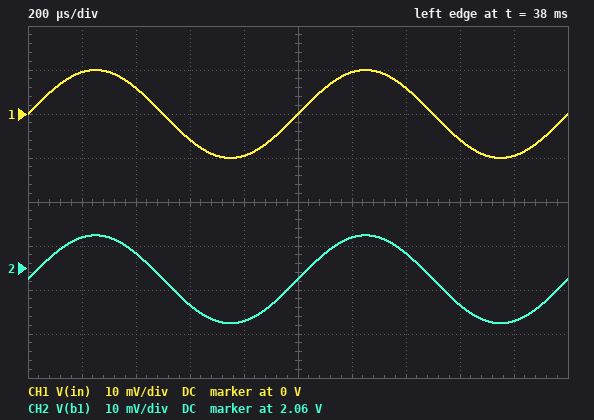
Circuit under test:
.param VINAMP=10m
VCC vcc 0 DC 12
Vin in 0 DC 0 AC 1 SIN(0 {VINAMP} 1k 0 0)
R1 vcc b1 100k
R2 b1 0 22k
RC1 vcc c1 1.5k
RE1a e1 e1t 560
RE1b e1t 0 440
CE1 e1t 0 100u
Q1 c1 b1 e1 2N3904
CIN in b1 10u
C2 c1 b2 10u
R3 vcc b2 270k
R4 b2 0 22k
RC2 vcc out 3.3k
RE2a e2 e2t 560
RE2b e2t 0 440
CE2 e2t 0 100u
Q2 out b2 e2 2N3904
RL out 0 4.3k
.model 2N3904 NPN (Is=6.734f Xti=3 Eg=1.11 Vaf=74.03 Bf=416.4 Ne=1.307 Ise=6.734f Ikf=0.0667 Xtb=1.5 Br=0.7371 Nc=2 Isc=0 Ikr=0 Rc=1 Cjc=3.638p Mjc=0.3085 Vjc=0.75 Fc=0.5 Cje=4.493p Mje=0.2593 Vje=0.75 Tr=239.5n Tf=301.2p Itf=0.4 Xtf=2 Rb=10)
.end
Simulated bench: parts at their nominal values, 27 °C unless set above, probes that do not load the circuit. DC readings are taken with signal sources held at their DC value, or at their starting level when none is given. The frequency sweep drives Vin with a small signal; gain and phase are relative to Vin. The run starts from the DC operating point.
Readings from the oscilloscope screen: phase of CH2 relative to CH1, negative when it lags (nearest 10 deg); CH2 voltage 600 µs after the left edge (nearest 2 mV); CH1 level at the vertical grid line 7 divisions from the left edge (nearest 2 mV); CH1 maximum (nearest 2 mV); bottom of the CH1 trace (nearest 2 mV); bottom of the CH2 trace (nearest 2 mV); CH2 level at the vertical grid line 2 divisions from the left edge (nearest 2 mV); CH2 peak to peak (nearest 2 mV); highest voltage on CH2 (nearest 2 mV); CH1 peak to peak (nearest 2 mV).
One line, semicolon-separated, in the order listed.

0 deg; 2.052 V; 6 mV; 10 mV; -10 mV; 2.048 V; 2.064 V; 20 mV; 2.068 V; 20 mV
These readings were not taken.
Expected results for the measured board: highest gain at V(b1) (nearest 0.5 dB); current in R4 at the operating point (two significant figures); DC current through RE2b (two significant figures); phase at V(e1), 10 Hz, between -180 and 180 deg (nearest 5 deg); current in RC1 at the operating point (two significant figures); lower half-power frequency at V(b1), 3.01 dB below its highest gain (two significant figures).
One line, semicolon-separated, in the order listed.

0 dB; 40 µA; 250 µA; 5 deg; 1.4 mA; 950 mHz
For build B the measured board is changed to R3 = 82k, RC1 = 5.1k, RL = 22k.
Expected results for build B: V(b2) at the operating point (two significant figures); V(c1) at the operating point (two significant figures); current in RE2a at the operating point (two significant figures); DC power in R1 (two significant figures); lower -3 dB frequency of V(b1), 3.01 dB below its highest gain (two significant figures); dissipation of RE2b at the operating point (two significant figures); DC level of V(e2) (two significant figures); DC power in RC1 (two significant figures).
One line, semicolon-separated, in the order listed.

2.4 V; 5.0 V; 1.7 mA; 990 µW; 960 mHz; 1.3 mW; 1.7 V; 9.6 mW
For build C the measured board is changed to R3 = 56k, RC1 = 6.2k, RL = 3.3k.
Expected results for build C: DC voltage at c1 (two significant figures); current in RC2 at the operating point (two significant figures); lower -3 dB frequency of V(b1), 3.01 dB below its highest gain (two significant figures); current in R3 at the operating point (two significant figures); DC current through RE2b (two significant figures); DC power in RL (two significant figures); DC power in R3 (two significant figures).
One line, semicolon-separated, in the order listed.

3.5 V; 2.9 mA; 960 mHz; 160 µA; 2.2 mA; 1.7 mW; 1.5 mW
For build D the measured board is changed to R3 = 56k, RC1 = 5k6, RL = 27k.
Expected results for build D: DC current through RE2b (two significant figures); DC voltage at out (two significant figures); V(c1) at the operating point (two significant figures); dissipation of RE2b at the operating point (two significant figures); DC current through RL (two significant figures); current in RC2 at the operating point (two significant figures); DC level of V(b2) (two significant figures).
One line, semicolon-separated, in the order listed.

2.5 mA; 3.3 V; 4.3 V; 2.8 mW; 120 µA; 2.6 mA; 3.2 V
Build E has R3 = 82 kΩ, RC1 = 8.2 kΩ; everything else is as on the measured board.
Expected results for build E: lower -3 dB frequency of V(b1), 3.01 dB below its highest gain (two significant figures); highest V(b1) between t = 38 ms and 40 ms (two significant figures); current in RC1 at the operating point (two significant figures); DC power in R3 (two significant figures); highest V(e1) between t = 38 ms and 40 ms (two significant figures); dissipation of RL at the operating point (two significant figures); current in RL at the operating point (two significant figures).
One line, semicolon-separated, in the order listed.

17 Hz; 2.0 V; 1.3 mA; 1.1 mW; 1.3 V; 3.0 mW; 830 µA
